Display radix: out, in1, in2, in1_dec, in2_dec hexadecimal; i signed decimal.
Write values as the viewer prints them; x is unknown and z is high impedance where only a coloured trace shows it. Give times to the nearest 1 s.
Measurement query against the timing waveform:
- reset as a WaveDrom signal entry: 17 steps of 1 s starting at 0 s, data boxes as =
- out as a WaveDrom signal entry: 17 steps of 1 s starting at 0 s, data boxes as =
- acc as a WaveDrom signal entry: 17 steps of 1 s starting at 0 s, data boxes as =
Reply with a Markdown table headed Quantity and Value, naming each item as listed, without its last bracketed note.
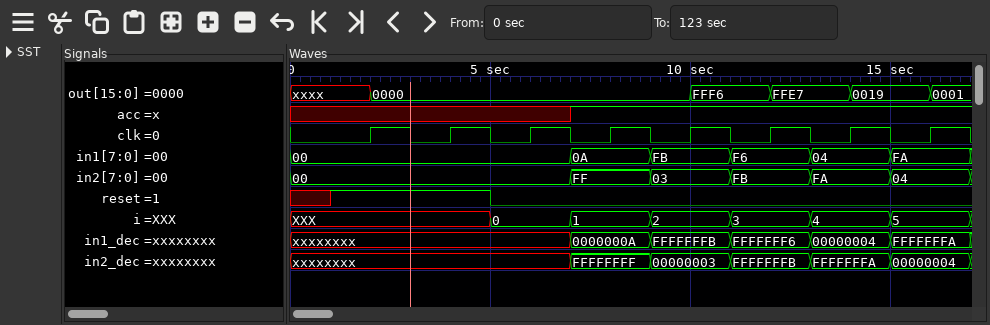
| Quantity | Value |
|---|---|
| reset as a WaveDrom signal entry: 17 steps of 1 s starting at 0 s, data boxes as = | {name: 'reset', wave: 'x1...0...........'} |
| out as a WaveDrom signal entry: 17 steps of 1 s starting at 0 s, data boxes as = | {name: 'out', wave: 'x.=.......=.=.=.=', data: '0000 FFF6 FFE7 0019 0001'} |
| acc as a WaveDrom signal entry: 17 steps of 1 s starting at 0 s, data boxes as = | {name: 'acc', wave: 'x......1.........'} |
